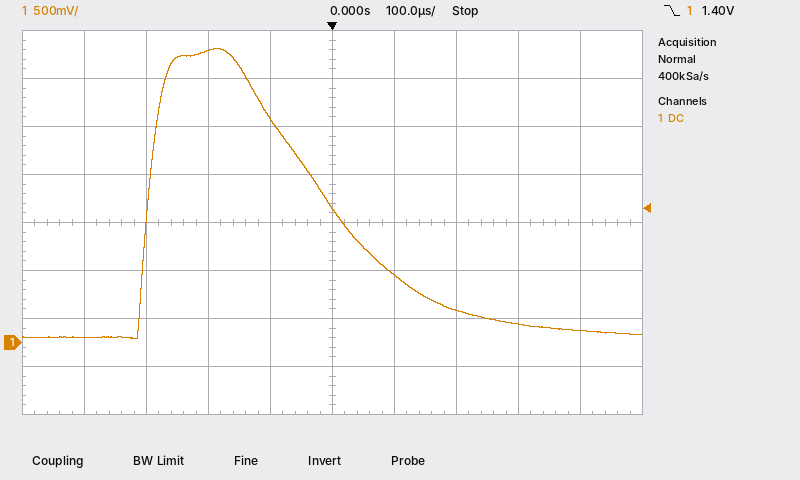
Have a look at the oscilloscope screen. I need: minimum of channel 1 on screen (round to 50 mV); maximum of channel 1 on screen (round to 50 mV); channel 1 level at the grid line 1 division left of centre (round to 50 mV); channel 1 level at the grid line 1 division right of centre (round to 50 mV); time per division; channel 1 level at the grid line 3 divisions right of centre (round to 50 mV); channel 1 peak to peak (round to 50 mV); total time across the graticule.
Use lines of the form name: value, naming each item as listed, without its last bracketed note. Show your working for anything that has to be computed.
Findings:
minimum of channel 1 on screen: 50 mV
maximum of channel 1 on screen: 3.05 V
channel 1 level at the grid line 1 division left of centre: 2.35 V
channel 1 level at the grid line 1 division right of centre: 700 mV
time per division: 100 µs
channel 1 level at the grid line 3 divisions right of centre: 200 mV
channel 1 peak to peak: 3.05 V − (50 mV) = 3.00 V
total time across the graticule: 1 ms
